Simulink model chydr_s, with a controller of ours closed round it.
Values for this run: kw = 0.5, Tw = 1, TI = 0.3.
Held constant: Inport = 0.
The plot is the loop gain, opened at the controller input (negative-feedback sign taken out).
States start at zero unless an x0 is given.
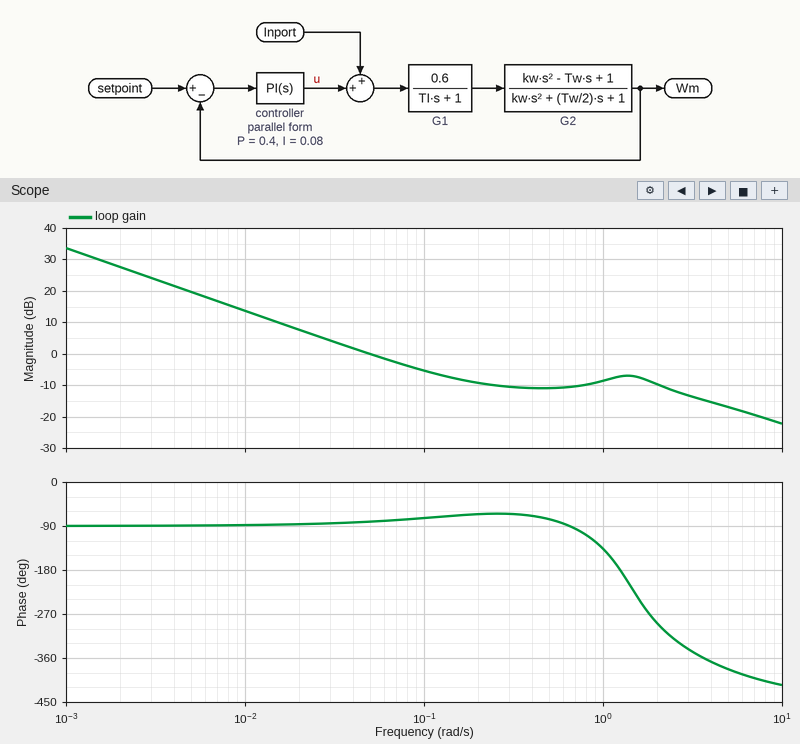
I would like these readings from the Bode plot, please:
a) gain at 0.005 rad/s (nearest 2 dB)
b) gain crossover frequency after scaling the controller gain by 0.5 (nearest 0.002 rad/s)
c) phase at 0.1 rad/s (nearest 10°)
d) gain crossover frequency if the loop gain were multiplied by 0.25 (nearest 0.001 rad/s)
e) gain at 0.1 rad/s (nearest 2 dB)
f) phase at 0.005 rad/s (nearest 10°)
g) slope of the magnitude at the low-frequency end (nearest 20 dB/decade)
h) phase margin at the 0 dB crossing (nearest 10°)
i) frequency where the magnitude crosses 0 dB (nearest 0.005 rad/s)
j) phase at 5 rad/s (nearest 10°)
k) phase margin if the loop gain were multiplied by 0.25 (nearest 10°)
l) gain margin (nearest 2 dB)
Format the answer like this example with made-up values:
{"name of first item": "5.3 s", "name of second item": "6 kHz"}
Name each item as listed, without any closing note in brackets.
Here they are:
{"gain at 0.005 rad/s": "20 dB", "gain crossover frequency after scaling the controller gain by 0.5": "0.024 rad/s", "phase at 0.1 rad/s": "-70°", "gain crossover frequency if the loop gain were multiplied by 0.25": "0.012 rad/s", "gain at 0.1 rad/s": "-6 dB", "phase at 0.005 rad/s": "-90°", "slope of the magnitude at the low-frequency end": "-20 dB/decade", "phase margin at the 0 dB crossing": "100°", "frequency where the magnitude crosses 0 dB": "0.050 rad/s", "phase at 5 rad/s": "-380°", "phase margin if the loop gain were multiplied by 0.25": "90°", "gain margin": "8 dB"}
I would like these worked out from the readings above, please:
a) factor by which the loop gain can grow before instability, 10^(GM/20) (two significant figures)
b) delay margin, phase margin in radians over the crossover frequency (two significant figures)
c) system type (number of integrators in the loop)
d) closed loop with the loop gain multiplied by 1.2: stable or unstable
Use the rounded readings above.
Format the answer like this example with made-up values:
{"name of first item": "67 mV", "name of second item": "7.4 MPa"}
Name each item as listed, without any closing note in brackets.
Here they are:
{"factor by which the loop gain can grow before instability, 10^(GM/20)": "2.5", "delay margin, phase margin in radians over the crossover frequency": "35 s", "system type": "1", "closed loop with the loop gain multiplied by 1.2: stable or unstable": "stable"}
